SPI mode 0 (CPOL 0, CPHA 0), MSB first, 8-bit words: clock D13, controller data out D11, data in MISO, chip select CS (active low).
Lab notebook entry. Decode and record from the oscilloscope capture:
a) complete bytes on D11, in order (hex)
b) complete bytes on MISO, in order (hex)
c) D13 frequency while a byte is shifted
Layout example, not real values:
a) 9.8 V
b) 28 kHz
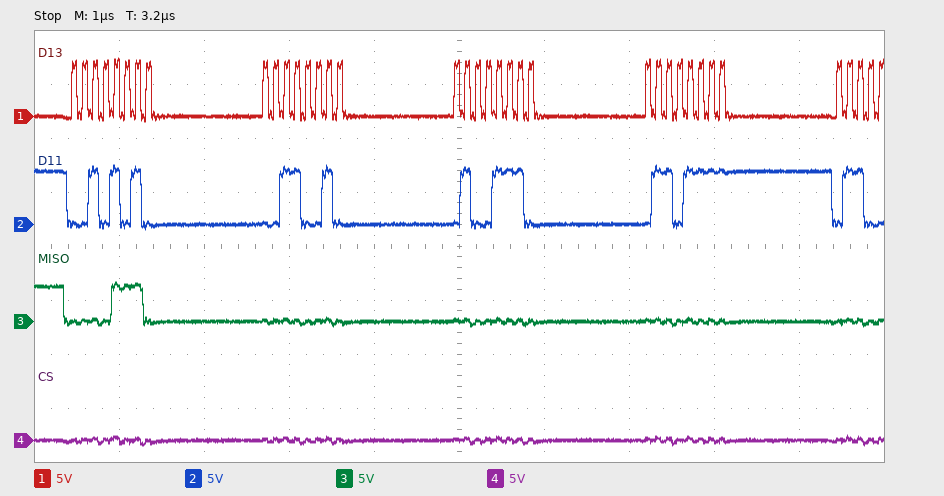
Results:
a) 0x2A 0x32 0x4E 0x6F
b) 0x0E 0x00 0x00 0x00
c) 8 MHz
